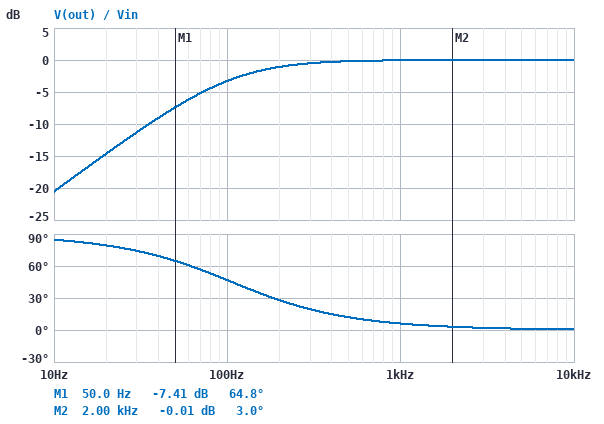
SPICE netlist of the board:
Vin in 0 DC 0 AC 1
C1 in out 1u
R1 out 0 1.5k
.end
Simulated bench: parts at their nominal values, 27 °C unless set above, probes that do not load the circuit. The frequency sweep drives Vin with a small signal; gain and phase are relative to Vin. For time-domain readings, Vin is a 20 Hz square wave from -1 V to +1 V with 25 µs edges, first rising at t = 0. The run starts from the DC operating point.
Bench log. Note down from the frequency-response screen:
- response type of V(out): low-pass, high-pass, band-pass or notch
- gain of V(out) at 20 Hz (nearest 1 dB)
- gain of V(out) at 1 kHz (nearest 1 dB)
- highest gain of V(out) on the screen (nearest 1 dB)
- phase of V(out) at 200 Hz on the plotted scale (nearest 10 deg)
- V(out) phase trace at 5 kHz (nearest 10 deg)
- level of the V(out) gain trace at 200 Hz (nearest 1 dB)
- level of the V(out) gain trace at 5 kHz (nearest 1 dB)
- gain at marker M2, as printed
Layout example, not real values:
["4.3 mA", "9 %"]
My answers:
["high-pass", "-15 dB", "0 dB", "0 dB", "30 deg", "0 deg", "-1 dB", "0 dB", "-0.01 dB"]
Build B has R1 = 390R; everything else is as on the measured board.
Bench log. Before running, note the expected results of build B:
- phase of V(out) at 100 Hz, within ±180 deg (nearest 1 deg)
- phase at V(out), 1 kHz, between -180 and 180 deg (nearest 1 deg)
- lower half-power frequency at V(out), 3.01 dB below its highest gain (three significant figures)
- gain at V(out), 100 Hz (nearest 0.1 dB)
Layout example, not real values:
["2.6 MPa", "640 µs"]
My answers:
["76 deg", "22 deg", "408 Hz", "-12.5 dB"]
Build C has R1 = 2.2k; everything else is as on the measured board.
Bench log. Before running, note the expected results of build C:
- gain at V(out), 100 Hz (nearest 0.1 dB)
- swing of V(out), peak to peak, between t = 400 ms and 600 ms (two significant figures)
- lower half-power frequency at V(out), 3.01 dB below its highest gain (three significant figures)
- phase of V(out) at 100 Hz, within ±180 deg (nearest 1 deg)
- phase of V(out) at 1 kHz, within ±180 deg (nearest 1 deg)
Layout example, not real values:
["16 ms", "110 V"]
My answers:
["-1.8 dB", "4.0 V", "72.3 Hz", "36 deg", "4 deg"]
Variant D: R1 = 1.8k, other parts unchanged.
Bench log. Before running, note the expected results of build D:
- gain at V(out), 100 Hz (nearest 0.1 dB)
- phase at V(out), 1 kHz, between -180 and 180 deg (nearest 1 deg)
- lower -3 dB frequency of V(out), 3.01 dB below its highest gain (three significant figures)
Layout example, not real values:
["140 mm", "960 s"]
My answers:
["-2.5 dB", "5 deg", "88.4 Hz"]
